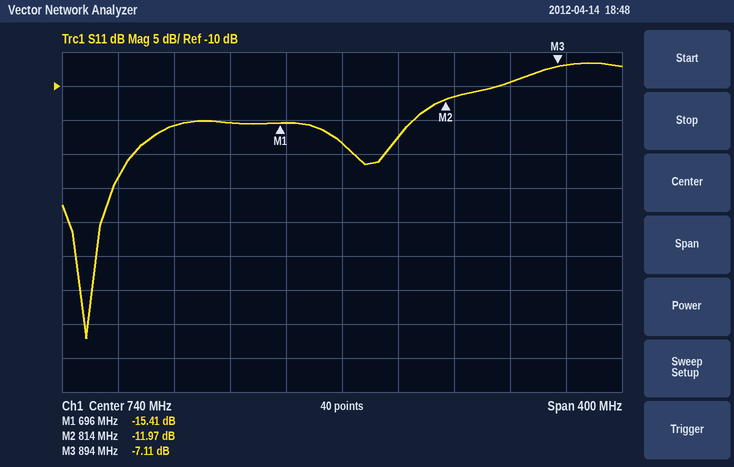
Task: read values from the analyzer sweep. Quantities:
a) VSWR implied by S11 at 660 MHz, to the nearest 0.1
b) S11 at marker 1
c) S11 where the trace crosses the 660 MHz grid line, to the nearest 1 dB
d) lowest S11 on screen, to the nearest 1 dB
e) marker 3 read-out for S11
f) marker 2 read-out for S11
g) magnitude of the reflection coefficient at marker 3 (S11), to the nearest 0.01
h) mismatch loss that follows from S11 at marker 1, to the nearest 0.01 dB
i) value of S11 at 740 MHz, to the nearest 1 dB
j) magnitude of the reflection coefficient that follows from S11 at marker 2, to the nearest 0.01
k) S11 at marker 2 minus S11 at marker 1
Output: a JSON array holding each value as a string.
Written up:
["1.4", "-15.41 dB", "-15 dB", "-47 dB", "-7.11 dB", "-11.97 dB", "0.44", "0.13 dB", "-18 dB", "0.25", "3.44 dB"]
